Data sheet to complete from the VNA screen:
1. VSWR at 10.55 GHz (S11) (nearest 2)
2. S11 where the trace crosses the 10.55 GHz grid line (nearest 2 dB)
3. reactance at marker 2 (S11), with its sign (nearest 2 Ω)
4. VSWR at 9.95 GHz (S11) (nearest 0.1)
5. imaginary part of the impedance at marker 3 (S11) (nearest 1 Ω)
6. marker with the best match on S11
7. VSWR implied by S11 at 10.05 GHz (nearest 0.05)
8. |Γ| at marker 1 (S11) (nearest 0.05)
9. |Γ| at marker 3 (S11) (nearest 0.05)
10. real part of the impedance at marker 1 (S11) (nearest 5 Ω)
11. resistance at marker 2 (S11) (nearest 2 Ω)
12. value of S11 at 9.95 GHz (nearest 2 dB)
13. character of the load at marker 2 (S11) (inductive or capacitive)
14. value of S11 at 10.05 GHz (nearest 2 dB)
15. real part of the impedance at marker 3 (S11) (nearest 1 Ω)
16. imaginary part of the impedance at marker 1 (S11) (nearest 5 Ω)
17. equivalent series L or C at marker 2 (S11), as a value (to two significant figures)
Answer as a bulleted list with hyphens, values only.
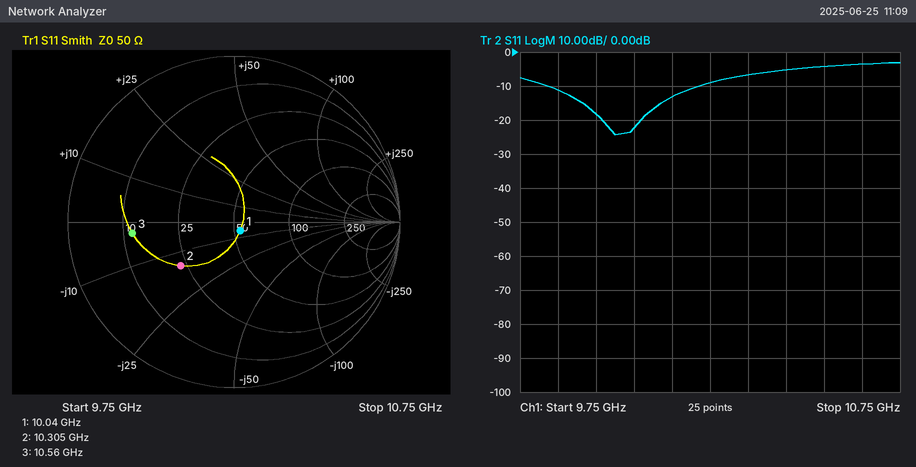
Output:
- 4
- -4 dB
- -14 Ω
- 1.3
- -3 Ω
- marker 1
- 1.15
- 0.05
- 0.60
- 55 Ω
- 22 Ω
- -18 dB
- capacitive
- -22 dB
- 12 Ω
- -5 Ω
- 1.1 pF
